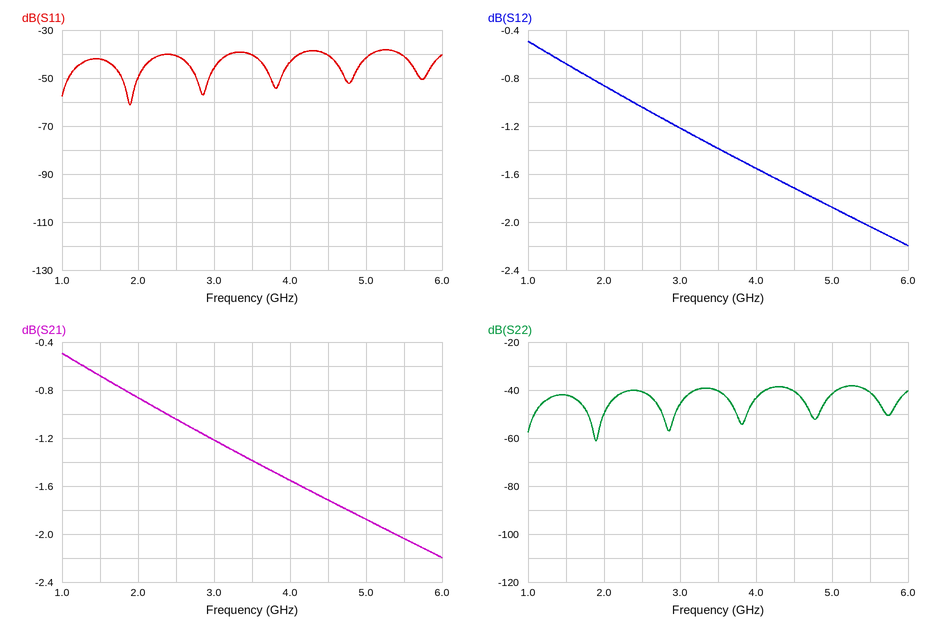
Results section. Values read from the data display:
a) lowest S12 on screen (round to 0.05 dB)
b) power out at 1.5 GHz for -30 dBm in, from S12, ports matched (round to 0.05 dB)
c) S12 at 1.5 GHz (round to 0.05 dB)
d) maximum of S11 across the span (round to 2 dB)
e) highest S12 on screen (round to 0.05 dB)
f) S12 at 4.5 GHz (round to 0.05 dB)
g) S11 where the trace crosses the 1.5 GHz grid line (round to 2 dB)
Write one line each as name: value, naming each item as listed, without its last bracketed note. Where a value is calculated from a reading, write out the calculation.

lowest S12 on screen: -2.20 dB
power out at 1.5 GHz for -30 dBm in, from S12, ports matched: -30 dBm + (-0.70 dB) = -30.70 dBm
S12 at 1.5 GHz: -0.70 dB
maximum of S11 across the span: -38 dB
highest S12 on screen: -0.50 dB
S12 at 4.5 GHz: -1.70 dB
S11 where the trace crosses the 1.5 GHz grid line: -42 dB
